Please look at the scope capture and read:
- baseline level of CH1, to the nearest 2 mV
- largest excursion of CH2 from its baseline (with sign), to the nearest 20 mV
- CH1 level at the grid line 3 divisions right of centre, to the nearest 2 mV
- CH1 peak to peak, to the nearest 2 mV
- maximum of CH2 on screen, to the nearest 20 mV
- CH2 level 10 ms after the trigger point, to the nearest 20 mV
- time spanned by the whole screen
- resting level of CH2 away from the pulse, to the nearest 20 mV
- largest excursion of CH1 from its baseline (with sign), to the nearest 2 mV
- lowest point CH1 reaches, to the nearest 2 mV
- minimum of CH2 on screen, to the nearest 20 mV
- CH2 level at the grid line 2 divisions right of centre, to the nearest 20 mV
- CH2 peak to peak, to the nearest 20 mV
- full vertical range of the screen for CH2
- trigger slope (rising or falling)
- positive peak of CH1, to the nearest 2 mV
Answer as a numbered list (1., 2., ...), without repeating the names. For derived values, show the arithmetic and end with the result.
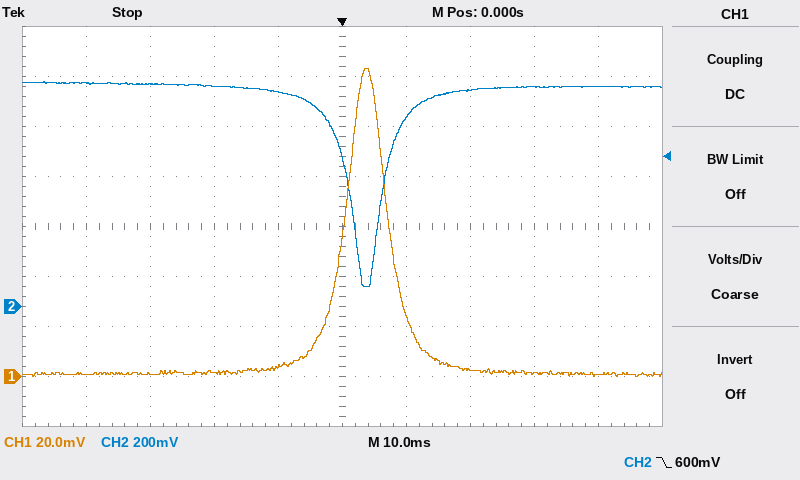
1. 2 mV
2. 80 mV − (880 mV) = -800 mV
3. 2 mV
4. 124 mV − (0 mV) = 124 mV
5. 900 mV
6. 760 mV
7. 100 ms
8. 880 mV
9. 124 mV − (2 mV) = +122 mV
10. 0 mV
11. 80 mV
12. 860 mV
13. 900 mV − (80 mV) = 820 mV
14. 1.6 V
15. falling
16. 124 mV
